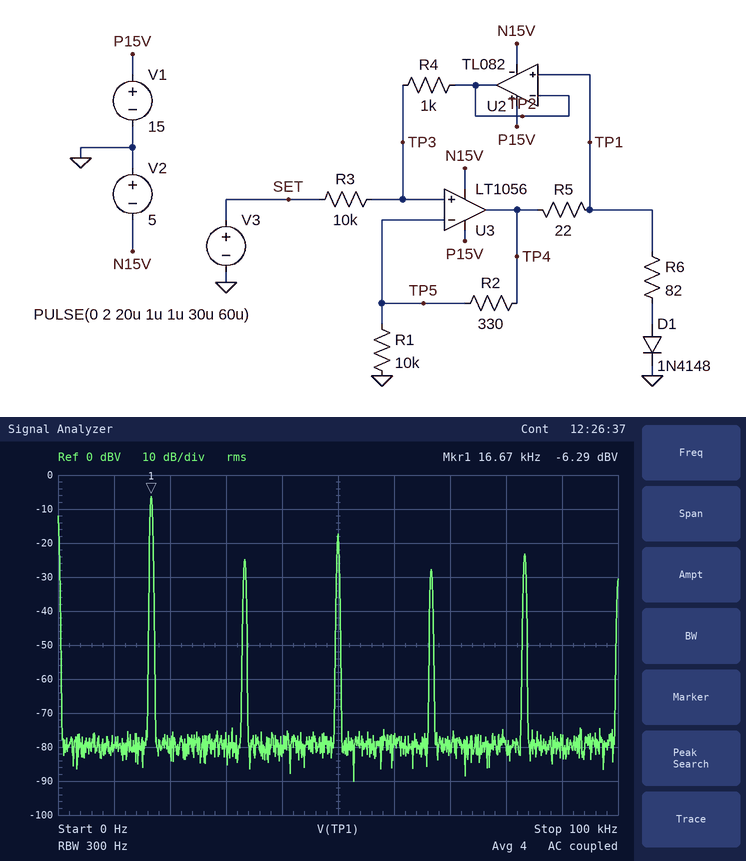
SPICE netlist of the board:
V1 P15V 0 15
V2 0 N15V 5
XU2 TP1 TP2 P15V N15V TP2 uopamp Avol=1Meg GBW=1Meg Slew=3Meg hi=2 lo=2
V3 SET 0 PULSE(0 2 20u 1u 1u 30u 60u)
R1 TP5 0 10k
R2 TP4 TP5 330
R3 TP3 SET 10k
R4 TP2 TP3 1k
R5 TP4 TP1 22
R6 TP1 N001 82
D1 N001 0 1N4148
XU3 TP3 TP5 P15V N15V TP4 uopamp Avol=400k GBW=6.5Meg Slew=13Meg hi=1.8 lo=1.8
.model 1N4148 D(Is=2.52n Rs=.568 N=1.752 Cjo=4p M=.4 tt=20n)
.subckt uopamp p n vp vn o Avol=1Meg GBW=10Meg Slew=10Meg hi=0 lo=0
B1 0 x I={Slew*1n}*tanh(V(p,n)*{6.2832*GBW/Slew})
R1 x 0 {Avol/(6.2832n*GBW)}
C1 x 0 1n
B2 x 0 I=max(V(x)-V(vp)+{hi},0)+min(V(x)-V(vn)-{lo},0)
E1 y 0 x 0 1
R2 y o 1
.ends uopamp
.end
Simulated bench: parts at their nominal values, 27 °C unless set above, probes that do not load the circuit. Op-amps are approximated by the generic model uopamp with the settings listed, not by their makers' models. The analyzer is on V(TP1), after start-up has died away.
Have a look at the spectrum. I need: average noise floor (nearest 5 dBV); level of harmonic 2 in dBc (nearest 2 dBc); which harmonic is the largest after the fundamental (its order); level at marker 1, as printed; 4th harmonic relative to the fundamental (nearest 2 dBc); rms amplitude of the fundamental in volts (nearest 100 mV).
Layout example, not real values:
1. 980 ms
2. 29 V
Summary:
1. -80 dBV
2. -18 dBc
3. 3
4. -6.29 dBV
5. -22 dBc
6. 500 mV
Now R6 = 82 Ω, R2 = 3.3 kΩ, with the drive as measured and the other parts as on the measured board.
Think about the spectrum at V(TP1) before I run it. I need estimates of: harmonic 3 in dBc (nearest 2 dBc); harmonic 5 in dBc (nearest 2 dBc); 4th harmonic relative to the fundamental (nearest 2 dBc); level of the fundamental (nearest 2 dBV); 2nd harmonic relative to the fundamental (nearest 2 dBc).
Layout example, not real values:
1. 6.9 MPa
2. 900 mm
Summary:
1. -10 dBc
2. -14 dBc
3. -26 dBc
4. -54 dBV
5. -26 dBc
